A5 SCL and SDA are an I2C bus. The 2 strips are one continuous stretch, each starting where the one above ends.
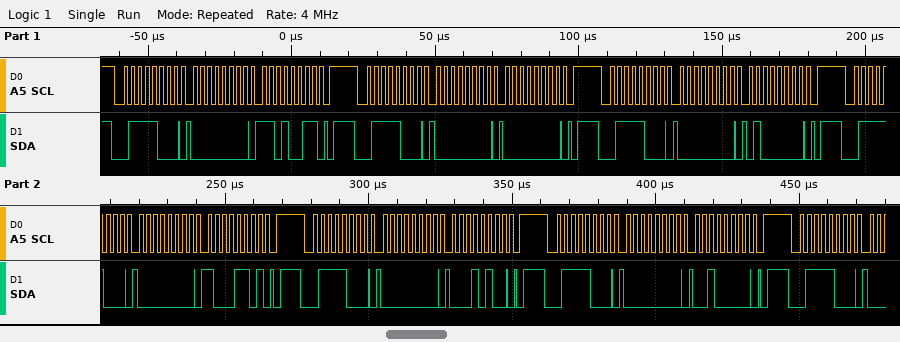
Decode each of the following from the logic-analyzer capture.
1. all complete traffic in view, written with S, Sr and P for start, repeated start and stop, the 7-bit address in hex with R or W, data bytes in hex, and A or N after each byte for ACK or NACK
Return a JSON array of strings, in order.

["S 3CW A 00 A D3 A P S 3CW A 00 A 00 A P S 3CW A 00 A 40 A P S 3CW A 00 A 8D A P S 3CW A 00 A 14 A P S 3CW A 00 A 20 A P S 3CW A"]
